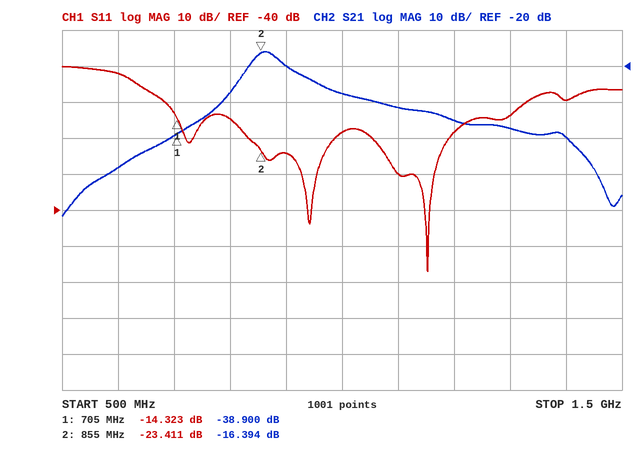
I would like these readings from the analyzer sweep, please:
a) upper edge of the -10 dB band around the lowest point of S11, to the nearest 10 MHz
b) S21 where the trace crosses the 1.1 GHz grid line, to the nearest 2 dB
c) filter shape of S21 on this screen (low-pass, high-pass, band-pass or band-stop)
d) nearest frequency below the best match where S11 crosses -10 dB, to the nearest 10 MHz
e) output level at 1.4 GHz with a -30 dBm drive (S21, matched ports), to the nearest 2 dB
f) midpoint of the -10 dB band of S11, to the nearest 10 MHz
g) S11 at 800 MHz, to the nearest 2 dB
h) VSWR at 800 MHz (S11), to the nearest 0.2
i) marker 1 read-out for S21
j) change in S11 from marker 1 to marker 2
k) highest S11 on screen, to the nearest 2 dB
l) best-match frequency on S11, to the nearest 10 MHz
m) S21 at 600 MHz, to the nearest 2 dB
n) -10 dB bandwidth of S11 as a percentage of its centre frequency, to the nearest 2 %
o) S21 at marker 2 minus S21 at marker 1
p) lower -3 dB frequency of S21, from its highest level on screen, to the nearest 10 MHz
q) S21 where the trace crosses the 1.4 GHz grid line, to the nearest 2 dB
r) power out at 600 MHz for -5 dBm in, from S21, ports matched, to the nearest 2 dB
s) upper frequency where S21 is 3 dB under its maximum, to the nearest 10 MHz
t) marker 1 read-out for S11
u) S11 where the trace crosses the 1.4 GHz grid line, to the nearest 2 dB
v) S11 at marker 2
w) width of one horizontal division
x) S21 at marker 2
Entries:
1.33 GHz
-32 dB
band-pass
680 MHz
-70 dBm
1.01 GHz
-14 dB
1.4
-38.900 dB
-9.088 dB
0 dB
1.15 GHz
-48 dB
64 %
22.506 dB
840 MHz
-40 dB
-54 dBm
890 MHz
-14.323 dB
-10 dB
-23.411 dB
100 MHz
-16.394 dB
